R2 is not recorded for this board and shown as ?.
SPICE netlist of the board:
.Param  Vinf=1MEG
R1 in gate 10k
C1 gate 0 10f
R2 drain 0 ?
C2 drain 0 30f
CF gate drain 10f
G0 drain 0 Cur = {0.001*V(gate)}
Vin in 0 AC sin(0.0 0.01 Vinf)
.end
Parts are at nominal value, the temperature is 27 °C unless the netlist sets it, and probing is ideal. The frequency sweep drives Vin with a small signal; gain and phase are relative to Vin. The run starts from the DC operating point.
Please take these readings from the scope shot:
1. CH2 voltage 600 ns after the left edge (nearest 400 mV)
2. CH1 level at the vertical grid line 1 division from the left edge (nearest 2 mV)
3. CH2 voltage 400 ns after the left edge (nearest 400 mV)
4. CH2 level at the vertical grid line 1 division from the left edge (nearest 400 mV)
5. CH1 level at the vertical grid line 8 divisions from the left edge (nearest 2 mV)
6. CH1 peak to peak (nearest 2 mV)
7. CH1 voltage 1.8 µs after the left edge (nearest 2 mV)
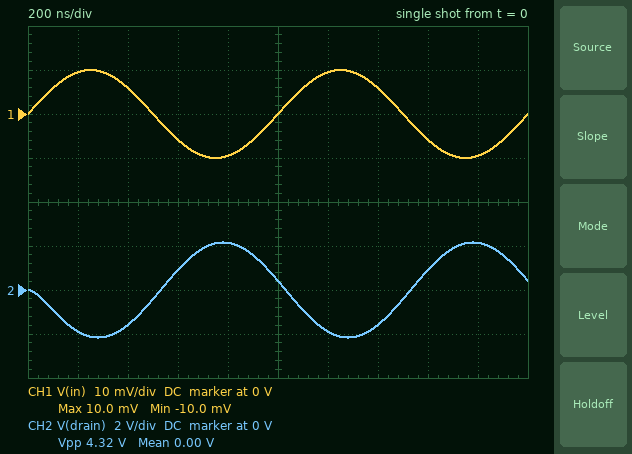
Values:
800 mV
10 mV
-1.6 V
-2.0 V
-6 mV
20 mV
-10 mV
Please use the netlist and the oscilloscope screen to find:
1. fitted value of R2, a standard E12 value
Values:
220 kΩ
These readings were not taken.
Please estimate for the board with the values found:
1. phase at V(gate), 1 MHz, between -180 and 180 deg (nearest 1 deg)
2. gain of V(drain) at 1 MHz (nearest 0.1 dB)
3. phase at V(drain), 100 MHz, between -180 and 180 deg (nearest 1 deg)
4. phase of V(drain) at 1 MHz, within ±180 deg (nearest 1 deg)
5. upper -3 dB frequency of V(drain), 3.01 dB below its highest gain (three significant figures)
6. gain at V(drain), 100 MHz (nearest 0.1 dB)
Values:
-8 deg
46.7 dB
91 deg
169 deg
5.14 MHz
21.1 dB
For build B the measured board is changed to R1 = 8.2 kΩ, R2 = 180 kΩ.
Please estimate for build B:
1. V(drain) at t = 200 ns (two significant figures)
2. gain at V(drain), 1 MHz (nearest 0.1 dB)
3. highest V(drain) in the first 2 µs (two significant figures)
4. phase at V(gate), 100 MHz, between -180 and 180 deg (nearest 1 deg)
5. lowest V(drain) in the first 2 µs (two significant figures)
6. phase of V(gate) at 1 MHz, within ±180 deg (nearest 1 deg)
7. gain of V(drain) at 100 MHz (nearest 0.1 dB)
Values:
-1.6 V
45.0 dB
1.8 V
-10 deg
-1.8 V
-5 deg
22.2 dB
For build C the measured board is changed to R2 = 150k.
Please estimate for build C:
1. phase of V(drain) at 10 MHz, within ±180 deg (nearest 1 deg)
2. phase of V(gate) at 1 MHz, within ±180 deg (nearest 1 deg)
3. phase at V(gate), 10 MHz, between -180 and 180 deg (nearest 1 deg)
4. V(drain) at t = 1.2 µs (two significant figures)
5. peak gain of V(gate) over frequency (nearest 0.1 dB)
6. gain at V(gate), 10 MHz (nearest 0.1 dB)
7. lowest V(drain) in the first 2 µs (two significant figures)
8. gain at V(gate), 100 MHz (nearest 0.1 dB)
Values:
127 deg
-5 deg
-33 deg
-1.3 V
0 dB
-3.8 dB
-1.5 V
-10.7 dB
